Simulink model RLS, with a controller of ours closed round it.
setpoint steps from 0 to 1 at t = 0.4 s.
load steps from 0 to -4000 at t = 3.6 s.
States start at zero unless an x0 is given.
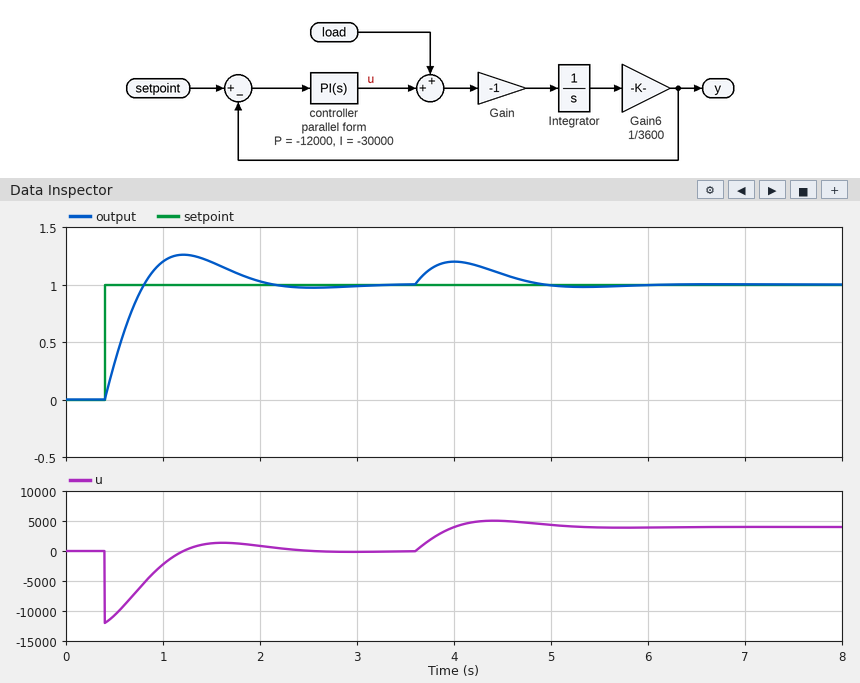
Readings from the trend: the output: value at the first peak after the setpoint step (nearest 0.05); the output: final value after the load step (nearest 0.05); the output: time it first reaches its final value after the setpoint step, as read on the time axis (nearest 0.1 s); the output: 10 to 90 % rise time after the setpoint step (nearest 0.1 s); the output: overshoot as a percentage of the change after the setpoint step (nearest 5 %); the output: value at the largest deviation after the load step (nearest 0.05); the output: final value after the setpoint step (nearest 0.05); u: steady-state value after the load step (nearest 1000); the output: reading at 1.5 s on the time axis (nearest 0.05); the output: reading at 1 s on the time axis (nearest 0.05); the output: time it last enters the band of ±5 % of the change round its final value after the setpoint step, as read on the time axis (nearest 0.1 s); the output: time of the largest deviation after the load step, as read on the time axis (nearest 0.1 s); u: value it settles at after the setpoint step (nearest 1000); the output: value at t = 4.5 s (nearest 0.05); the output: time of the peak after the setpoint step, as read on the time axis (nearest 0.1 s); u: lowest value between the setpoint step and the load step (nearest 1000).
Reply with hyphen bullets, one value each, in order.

- 1.25
- 1.00
- 0.8 s
- 0.3 s
- 25 %
- 1.20
- 1.00
- 4000
- 1.20
- 1.20
- 1.9 s
- 4.0 s
- 0
- 1.10
- 1.2 s
- -12000
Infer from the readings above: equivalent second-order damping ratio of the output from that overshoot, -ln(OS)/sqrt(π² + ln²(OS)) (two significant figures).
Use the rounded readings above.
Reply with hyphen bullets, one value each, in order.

- 0.40
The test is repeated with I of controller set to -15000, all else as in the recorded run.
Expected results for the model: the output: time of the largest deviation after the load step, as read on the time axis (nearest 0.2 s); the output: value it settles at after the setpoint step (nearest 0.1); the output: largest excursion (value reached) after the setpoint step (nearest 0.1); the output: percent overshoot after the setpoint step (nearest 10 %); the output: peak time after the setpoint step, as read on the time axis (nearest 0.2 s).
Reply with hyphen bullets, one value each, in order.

- 4.2 s
- 1.0
- 1.2
- 20 %
- 1.4 s
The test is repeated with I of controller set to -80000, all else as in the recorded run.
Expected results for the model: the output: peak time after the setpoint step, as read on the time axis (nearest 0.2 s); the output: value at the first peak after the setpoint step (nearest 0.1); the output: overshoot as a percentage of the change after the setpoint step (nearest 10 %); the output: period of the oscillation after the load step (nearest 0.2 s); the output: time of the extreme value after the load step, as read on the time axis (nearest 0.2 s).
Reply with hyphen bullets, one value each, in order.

- 1.0 s
- 1.4
- 40 %
- 1.4 s
- 3.8 s
